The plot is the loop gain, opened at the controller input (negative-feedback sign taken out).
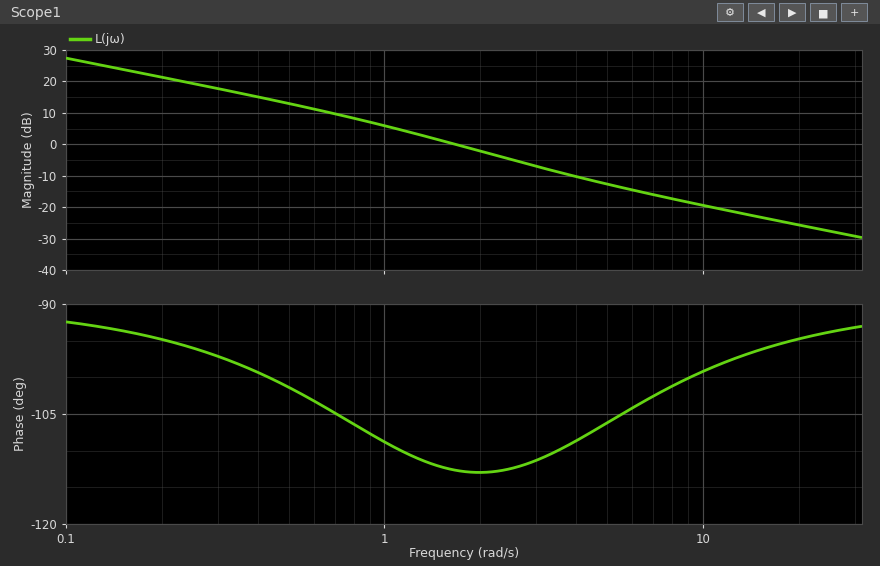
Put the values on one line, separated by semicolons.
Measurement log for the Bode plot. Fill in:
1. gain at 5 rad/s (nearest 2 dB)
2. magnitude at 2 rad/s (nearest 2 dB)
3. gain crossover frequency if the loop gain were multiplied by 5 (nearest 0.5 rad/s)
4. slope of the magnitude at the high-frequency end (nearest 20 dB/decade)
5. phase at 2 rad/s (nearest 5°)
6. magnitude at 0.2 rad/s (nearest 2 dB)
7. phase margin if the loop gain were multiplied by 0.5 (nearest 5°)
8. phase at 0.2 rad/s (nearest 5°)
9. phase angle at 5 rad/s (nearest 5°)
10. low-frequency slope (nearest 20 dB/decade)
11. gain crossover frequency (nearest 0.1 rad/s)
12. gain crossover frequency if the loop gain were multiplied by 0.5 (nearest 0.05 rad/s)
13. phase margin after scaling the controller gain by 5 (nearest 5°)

-12 dB; -2 dB; 5.5 rad/s; -20 dB/decade; -115°; 22 dB; 70°; -95°; -105°; -20 dB/decade; 1.7 rad/s; 1.00 rad/s; 75°
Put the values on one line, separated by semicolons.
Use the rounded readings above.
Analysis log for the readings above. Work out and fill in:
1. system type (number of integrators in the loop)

1
